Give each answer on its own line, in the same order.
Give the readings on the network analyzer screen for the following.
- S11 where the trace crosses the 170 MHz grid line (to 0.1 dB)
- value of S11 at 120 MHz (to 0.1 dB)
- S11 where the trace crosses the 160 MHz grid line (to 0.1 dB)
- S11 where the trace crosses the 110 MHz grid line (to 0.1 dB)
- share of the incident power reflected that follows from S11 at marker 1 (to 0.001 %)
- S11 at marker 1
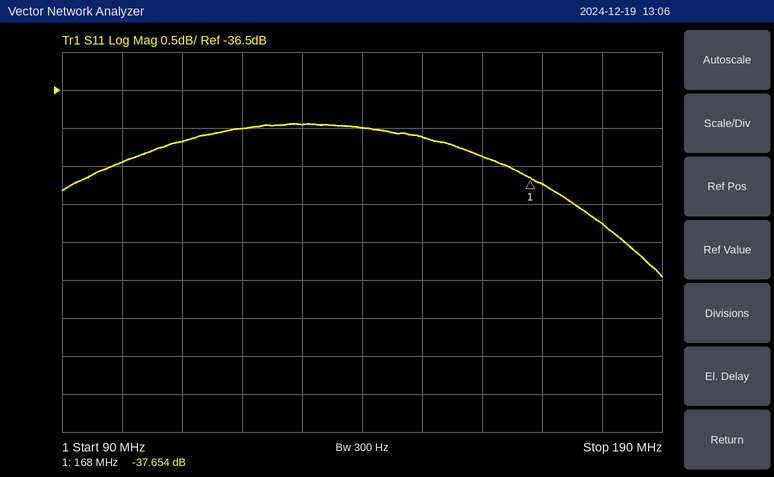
-37.7 dB
-37.0 dB
-37.4 dB
-37.2 dB
0.017 %
-37.654 dB
